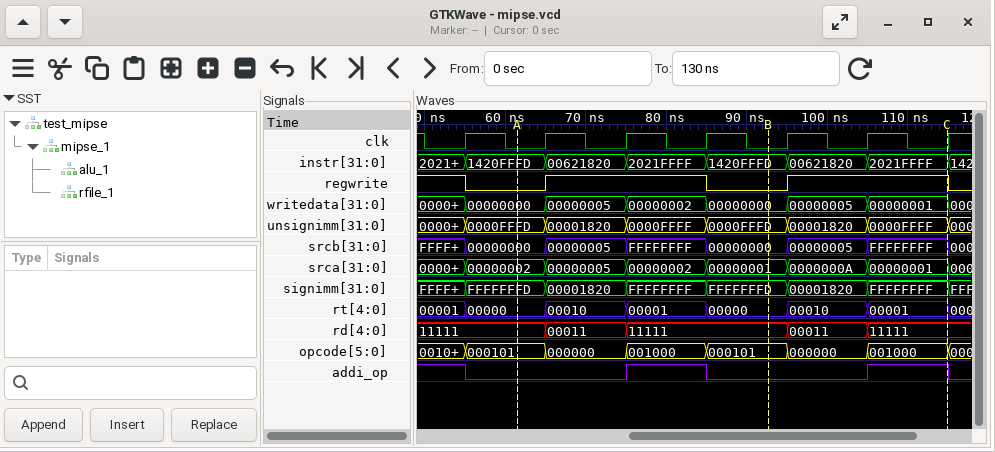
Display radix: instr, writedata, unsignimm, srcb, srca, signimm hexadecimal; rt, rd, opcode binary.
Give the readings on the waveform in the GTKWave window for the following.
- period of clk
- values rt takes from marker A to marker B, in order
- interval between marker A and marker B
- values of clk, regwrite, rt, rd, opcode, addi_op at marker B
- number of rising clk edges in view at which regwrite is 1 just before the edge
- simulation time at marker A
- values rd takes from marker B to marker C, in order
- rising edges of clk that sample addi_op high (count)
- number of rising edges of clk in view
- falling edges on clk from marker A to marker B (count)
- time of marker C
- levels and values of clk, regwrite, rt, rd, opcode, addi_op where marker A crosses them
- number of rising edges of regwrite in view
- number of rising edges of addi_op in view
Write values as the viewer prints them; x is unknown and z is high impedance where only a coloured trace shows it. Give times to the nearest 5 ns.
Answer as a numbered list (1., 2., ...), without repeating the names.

1. 10 ns
2. 00000, 00010, 00001, 00000
3. 30 ns
4. clk=0, regwrite=0, rt=00000, rd=11111, opcode=000101, addi_op=0
5. 5
6. 60 ns
7. 11111, 00011, 11111
8. 3
9. 7
10. 3
11. 115 ns
12. clk=0, regwrite=0, rt=00000, rd=11111, opcode=000101, addi_op=0
13. 2
14. 2
